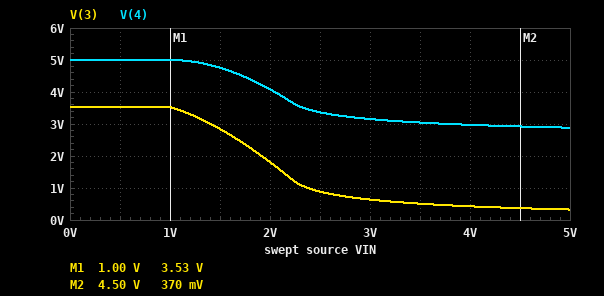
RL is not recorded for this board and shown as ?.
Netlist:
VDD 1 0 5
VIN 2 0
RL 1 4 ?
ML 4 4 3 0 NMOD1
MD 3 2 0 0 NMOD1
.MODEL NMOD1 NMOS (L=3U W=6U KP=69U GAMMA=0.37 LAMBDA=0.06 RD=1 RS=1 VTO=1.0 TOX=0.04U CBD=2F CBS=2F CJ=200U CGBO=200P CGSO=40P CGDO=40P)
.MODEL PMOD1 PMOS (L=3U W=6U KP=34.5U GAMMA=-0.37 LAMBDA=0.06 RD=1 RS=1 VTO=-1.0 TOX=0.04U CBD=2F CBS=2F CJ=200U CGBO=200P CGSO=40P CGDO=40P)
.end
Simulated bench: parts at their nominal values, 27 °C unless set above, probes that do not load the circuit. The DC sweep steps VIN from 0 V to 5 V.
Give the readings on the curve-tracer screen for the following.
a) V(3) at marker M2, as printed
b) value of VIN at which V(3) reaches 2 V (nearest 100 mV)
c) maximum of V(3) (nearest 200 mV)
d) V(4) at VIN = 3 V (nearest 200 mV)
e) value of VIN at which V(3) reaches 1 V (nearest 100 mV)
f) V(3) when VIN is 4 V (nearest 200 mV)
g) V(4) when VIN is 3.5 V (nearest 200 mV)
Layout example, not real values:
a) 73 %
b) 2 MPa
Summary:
a) 370 mV
b) 1.9 V
c) 3.6 V
d) 3.2 V
e) 2.4 V
f) 400 mV
g) 3.0 V
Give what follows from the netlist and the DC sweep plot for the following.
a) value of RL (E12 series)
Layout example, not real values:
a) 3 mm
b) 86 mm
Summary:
a) 12 kΩ
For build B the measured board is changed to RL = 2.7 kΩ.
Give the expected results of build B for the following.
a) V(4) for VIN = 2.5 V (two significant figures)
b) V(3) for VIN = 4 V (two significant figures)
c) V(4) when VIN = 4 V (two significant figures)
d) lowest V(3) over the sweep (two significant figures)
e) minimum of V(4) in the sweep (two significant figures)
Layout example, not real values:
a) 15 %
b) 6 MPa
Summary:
a) 4.5 V
b) 910 mV
c) 4.1 V
d) 720 mV
e) 4.0 V
